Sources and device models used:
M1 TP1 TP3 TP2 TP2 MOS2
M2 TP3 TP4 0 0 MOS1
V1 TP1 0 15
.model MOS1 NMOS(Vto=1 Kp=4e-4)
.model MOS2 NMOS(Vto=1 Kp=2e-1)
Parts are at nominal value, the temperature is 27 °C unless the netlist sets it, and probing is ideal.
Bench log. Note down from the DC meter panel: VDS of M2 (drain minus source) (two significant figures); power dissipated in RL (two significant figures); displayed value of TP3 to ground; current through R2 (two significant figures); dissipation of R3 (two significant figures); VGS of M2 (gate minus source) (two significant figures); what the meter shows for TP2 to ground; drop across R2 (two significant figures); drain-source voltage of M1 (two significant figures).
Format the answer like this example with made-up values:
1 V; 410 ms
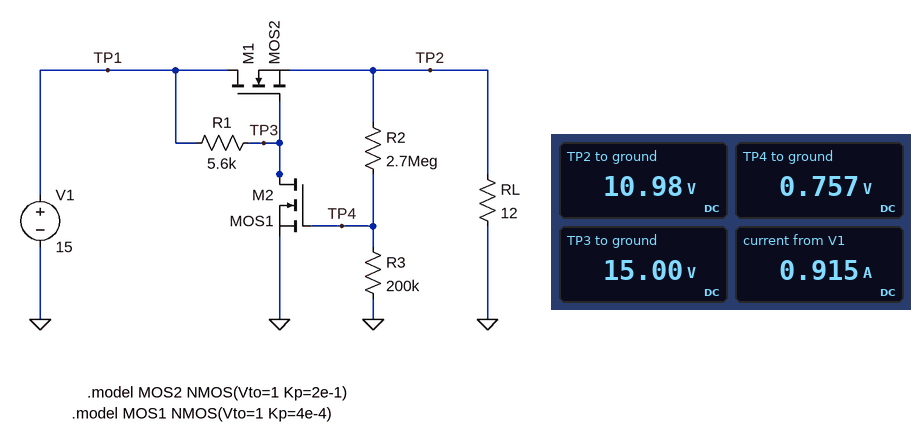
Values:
15 V; 10 W; 15.00 V; 3.8 µA; 2.9 µW; 760 mV; 10.98 V; 10 V; 4.0 V
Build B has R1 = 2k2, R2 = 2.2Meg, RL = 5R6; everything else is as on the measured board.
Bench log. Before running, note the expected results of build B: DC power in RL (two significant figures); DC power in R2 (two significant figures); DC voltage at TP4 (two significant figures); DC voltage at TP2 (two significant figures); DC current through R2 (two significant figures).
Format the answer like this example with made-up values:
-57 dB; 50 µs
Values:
17 W; 37 µW; 820 mV; 9.8 V; 4.1 µA
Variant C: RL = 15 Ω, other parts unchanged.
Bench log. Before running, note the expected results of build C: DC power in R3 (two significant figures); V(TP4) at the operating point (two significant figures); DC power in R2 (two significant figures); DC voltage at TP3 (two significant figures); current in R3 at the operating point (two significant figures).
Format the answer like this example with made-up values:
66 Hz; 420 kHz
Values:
3.0 µW; 780 mV; 41 µW; 15 V; 3.9 µA
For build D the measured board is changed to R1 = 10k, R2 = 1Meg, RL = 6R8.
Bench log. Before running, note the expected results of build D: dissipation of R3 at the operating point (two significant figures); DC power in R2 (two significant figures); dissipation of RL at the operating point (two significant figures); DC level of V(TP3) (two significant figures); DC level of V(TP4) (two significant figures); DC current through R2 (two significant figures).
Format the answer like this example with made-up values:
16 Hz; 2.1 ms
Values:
13 µW; 63 µW; 13 W; 14 V; 1.6 V; 8.0 µA
